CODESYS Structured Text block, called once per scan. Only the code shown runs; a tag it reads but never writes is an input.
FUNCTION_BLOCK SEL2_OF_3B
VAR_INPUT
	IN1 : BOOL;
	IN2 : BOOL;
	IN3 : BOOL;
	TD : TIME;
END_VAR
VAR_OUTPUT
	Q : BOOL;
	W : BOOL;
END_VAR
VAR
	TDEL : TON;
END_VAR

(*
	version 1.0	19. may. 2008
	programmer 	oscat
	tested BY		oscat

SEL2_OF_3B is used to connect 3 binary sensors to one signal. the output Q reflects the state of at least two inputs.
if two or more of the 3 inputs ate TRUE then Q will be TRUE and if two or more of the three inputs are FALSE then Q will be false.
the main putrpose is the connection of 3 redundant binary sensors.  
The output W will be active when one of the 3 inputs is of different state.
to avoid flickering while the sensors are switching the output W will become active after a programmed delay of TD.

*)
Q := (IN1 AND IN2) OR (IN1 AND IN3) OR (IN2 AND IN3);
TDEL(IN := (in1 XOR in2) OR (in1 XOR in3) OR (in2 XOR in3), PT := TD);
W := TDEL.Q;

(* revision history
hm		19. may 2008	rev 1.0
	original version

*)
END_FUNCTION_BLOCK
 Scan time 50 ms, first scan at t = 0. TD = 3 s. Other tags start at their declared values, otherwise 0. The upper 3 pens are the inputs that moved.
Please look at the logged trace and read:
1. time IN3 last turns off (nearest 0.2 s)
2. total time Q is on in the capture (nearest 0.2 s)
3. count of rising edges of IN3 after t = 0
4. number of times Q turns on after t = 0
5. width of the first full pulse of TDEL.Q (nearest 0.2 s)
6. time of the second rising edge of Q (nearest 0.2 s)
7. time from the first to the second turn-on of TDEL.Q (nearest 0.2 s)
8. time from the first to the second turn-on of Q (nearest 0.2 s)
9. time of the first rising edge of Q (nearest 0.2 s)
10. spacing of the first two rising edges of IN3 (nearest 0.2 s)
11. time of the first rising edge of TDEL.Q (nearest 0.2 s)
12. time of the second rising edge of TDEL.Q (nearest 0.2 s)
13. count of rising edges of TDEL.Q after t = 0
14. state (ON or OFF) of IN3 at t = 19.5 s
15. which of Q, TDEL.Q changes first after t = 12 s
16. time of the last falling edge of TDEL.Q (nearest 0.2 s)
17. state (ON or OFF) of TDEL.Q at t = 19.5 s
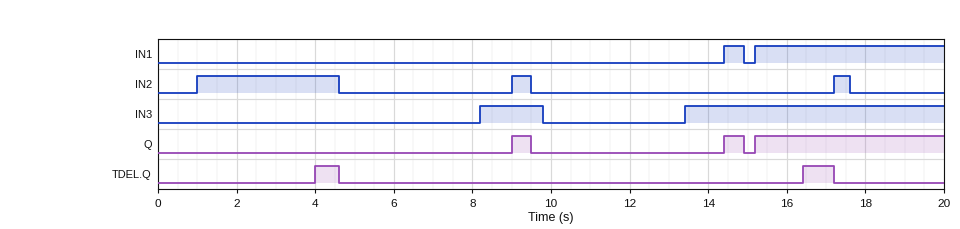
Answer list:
9.8 s
5.8 s
2
3
0.6 s
14.4 s
12.4 s
5.4 s
9.0 s
5.2 s
4.0 s
16.4 s
2
ON
Q
17.2 s
OFF
